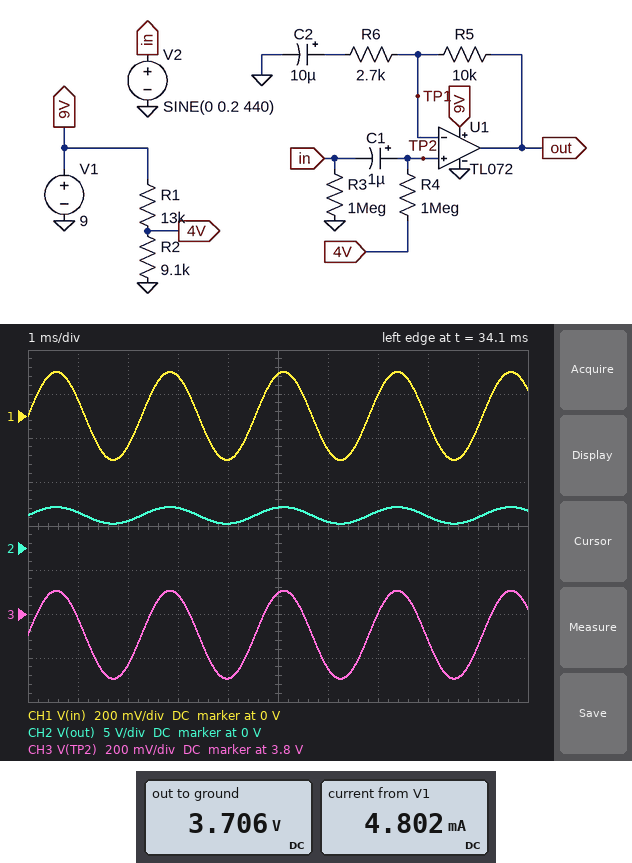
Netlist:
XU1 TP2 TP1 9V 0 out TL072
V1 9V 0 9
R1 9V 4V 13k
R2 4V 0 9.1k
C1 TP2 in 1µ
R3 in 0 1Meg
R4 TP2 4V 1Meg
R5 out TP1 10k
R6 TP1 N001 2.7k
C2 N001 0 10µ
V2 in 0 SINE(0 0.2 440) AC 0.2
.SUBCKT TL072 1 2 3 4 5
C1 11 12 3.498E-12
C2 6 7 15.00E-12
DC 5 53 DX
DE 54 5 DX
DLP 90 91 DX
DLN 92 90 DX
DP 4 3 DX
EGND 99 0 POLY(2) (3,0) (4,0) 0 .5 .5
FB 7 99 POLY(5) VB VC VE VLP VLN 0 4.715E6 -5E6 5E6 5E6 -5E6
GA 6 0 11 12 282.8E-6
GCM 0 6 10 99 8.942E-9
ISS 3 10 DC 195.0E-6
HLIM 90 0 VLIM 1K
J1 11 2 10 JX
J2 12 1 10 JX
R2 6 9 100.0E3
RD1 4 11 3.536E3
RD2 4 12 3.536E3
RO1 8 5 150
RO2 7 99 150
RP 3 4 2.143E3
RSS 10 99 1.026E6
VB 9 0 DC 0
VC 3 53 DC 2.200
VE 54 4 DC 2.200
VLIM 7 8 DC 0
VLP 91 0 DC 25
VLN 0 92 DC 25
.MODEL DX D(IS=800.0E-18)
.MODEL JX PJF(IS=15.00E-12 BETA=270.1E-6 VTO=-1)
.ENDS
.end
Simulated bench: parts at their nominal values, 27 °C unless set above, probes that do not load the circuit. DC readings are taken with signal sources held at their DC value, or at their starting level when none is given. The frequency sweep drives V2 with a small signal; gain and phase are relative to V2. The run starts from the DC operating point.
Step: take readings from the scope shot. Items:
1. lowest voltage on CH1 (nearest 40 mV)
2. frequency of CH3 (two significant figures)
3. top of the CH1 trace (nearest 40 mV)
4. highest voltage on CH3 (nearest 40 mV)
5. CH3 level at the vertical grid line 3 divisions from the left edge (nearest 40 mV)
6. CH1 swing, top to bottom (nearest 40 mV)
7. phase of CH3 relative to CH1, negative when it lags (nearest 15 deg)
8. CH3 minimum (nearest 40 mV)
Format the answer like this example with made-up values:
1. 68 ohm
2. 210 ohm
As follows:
1. -200 mV
2. 440 Hz
3. 200 mV
4. 3.92 V
5. 3.88 V
6. 400 mV
7. 0 deg
8. 3.52 V
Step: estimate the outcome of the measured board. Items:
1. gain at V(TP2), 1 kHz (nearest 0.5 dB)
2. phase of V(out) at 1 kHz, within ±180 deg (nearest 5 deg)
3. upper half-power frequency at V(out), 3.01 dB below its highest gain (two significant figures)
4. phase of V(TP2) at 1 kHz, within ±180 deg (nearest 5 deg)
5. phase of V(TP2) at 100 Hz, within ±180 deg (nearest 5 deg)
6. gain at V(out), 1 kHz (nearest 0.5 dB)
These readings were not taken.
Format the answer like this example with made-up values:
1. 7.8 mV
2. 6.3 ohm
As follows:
1. 0 dB
2. 0 deg
3. 820 kHz
4. 0 deg
5. 0 deg
6. 13.5 dB
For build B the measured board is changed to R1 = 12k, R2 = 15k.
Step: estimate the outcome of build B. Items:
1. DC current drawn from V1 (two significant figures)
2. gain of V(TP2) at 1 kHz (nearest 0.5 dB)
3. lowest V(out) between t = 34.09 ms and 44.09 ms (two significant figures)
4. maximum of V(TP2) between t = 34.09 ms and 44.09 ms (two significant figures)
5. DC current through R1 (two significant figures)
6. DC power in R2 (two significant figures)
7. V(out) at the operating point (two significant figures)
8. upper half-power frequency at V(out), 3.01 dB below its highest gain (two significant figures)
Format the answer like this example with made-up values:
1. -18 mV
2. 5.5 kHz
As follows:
1. 4.7 mA
2. 0 dB
3. 4.1 V
4. 5.2 V
5. 330 µA
6. 1.7 mW
7. 5.0 V
8. 810 kHz
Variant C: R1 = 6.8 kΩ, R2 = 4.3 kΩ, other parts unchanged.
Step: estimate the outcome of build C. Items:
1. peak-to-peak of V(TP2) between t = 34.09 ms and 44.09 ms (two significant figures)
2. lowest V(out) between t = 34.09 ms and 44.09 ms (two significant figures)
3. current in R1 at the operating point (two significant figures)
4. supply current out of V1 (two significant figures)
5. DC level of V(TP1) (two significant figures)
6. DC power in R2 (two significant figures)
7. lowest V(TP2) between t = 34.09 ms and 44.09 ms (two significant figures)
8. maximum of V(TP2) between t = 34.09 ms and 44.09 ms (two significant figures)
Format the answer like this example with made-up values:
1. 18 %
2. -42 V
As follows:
1. 400 mV
2. 2.5 V
3. 810 µA
4. 5.2 mA
5. 3.5 V
6. 2.8 mW
7. 3.3 V
8. 3.7 V
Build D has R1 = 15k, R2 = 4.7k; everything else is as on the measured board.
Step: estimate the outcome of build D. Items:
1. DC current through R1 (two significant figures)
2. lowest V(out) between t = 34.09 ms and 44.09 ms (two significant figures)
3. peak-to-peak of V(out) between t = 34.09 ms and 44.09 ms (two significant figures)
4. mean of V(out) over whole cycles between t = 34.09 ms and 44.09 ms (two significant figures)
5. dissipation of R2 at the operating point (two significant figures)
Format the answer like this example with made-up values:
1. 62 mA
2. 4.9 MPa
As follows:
1. 460 µA
2. 1.6 V
3. 1.5 V
4. 2.2 V
5. 980 µW
